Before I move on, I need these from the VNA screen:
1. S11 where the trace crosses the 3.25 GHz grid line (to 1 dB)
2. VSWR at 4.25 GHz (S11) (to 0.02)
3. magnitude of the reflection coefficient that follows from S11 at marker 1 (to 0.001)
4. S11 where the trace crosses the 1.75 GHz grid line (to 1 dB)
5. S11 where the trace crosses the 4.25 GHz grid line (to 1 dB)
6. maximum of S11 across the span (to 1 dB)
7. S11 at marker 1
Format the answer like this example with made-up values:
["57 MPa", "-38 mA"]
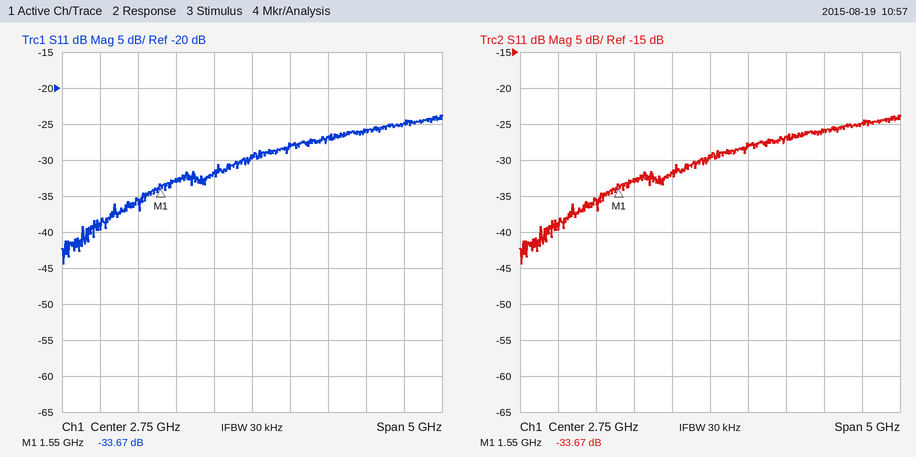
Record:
["-28 dB", "1.10", "0.021", "-33 dB", "-26 dB", "-24 dB", "-33.67 dB"]
